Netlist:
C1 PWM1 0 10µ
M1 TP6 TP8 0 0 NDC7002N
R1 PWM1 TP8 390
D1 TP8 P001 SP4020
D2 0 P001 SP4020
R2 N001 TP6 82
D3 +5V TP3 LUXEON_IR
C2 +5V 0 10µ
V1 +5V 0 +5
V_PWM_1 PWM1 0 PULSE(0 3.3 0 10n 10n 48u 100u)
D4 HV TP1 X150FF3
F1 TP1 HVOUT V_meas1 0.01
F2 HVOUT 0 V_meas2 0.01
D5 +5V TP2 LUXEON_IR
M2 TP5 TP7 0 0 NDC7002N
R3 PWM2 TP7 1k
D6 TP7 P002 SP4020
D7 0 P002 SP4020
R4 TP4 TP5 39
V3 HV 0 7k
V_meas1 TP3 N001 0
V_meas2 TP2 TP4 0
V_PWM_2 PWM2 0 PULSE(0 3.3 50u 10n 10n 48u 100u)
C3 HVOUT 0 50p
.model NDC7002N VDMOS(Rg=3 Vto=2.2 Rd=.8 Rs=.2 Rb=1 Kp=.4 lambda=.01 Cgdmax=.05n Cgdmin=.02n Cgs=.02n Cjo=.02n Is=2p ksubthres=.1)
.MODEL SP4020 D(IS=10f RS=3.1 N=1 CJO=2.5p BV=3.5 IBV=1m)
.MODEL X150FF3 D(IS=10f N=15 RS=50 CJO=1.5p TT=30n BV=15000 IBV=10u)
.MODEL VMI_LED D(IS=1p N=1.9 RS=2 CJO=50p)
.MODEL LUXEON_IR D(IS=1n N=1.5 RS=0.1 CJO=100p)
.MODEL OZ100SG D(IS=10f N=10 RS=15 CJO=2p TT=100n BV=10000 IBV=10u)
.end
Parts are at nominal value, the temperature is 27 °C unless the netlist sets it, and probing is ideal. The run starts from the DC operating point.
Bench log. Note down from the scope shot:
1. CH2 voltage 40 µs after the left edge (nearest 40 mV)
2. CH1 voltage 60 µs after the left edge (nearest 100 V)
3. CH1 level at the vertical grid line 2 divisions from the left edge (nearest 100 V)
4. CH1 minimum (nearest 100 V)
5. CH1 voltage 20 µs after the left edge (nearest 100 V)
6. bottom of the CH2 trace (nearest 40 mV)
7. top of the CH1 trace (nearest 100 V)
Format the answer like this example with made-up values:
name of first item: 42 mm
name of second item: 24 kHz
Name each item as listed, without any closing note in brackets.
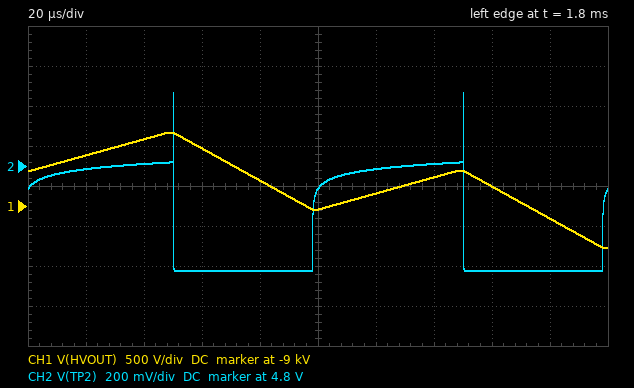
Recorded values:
CH2 voltage 40 µs after the left edge: 4.80 V
CH1 voltage 60 µs after the left edge: -8.3 kV
CH1 level at the vertical grid line 2 divisions from the left edge: -8.2 kV
CH1 minimum: -9.5 kV
CH1 voltage 20 µs after the left edge: -8.4 kV
bottom of the CH2 trace: 4.28 V
top of the CH1 trace: -8.1 kV
